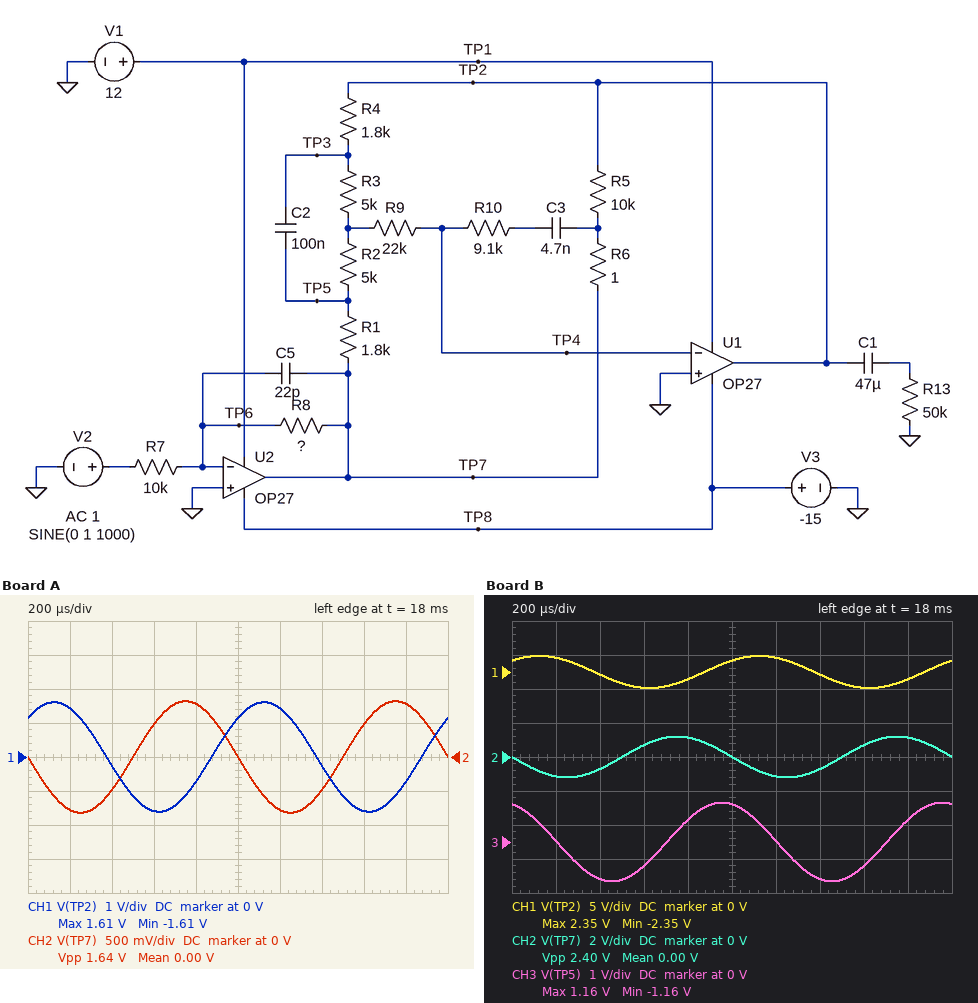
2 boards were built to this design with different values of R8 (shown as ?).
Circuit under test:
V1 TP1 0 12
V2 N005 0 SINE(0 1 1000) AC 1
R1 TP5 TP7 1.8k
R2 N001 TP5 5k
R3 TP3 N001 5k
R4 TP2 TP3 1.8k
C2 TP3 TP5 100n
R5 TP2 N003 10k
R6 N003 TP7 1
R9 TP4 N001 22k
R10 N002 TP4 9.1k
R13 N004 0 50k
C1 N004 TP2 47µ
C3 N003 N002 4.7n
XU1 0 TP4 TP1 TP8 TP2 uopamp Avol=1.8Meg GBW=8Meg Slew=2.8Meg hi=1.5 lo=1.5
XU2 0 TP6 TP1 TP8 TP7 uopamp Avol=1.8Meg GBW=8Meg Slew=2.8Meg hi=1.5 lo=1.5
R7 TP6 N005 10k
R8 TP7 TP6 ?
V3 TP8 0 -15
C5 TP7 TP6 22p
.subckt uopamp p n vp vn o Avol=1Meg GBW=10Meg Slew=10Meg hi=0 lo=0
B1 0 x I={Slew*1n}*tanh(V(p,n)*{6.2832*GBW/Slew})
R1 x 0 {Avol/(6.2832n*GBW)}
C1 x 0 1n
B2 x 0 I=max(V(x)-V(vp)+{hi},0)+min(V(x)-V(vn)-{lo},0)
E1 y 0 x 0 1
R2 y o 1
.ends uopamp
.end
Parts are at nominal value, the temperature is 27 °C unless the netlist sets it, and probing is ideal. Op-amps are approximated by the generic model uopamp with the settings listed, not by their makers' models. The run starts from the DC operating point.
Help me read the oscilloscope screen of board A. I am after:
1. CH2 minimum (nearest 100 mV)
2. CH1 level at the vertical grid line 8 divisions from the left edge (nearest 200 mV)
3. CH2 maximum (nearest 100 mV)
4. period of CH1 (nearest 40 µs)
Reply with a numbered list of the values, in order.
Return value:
1. -800 mV
2. -1.6 V
3. 800 mV
4. 1.00 ms
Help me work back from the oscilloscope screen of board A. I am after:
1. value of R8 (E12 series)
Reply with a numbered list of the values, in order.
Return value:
1. 8.2 kΩ
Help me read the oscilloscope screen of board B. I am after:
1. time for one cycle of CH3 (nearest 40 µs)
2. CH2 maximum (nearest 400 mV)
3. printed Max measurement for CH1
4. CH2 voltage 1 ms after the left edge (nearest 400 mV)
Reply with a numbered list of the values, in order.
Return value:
1. 1.00 ms
2. 1.2 V
3. 2.35 V
4. 0 V
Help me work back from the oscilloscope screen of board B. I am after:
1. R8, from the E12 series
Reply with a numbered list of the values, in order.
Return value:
1. 12 kΩ
